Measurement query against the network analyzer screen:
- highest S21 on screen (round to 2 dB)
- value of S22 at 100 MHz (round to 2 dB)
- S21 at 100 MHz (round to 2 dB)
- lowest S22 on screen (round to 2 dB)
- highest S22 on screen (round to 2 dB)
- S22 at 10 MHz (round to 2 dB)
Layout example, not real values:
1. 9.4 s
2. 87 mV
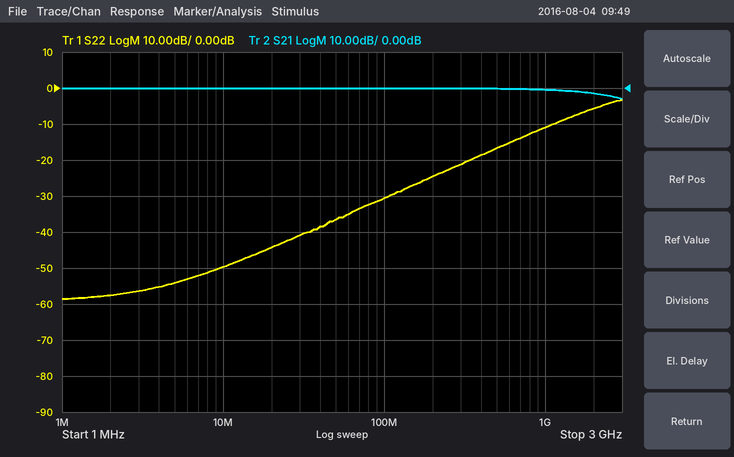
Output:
1. 0 dB
2. -30 dB
3. 0 dB
4. -58 dB
5. -4 dB
6. -50 dB
